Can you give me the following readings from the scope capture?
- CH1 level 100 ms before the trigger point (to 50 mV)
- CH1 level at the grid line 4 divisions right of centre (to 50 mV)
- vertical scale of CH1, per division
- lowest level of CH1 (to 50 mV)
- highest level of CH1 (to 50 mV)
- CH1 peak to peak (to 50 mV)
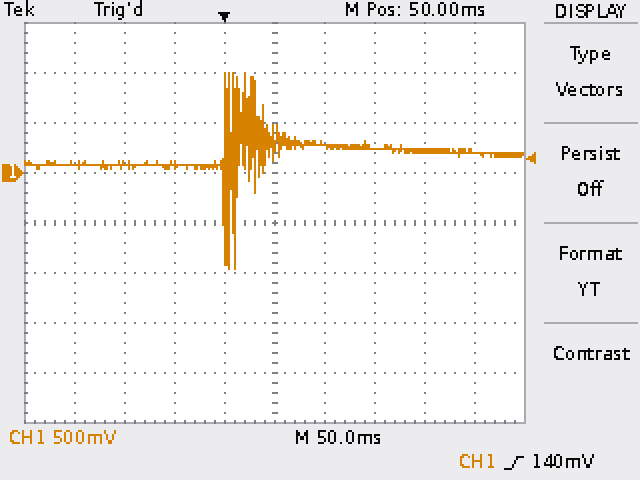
100 mV
200 mV
500 mV
-950 mV
1.00 V
1.95 V
